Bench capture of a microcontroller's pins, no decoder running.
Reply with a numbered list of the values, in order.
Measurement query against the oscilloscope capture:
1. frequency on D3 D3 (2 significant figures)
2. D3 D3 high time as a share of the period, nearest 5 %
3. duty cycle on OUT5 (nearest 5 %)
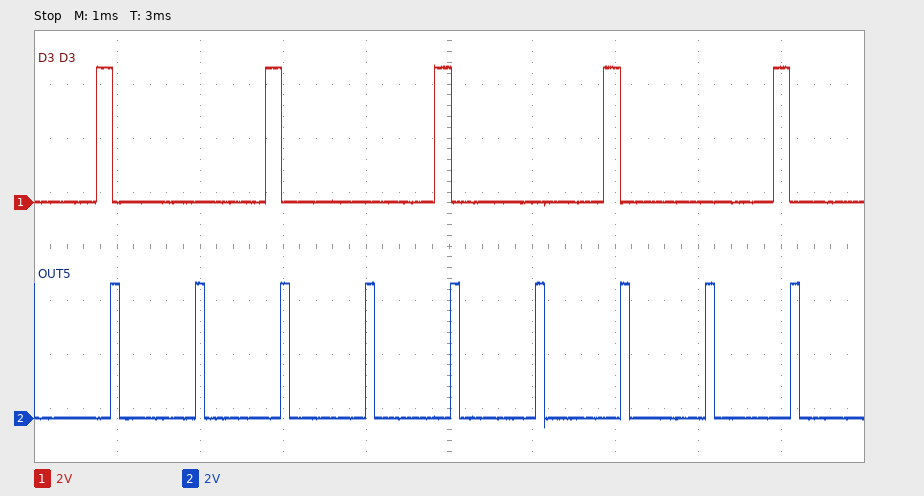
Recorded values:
1. 490 Hz
2. 10 %
3. 10 %
